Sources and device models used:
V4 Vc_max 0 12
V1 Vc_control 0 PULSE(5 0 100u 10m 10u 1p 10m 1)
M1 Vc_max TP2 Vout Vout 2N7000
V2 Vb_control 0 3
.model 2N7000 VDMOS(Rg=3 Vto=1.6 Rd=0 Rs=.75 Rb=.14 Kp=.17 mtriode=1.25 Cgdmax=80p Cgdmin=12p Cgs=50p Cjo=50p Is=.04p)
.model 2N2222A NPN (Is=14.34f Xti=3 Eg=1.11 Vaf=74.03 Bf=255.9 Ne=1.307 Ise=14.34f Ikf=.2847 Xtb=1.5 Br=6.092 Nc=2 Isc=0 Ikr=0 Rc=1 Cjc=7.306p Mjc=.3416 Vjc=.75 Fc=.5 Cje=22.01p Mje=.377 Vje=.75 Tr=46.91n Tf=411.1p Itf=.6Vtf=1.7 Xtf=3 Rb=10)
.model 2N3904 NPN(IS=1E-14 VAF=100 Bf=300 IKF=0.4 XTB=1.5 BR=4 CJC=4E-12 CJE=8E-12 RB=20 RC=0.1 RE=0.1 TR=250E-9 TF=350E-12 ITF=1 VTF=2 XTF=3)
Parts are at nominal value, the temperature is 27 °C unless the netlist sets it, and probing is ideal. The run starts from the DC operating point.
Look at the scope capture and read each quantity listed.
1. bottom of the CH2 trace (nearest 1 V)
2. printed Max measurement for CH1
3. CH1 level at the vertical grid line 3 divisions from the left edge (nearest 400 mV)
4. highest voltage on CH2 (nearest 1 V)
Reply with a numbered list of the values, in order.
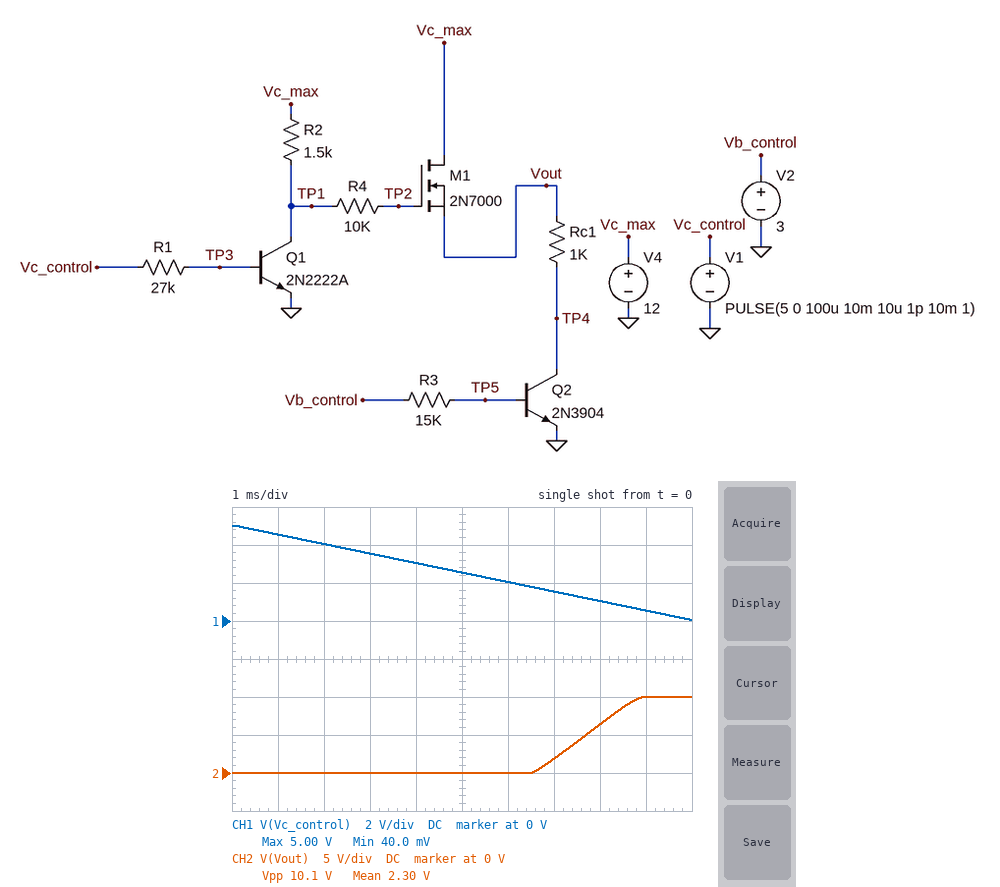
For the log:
1. 0 V
2. 5.00 V
3. 3.6 V
4. 10 V
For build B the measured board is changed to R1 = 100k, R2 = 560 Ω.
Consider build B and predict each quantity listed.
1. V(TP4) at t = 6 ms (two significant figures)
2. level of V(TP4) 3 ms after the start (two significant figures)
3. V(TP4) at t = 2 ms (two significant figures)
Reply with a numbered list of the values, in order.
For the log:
1. 79 mV
2. 72 mV
3. 70 mV
